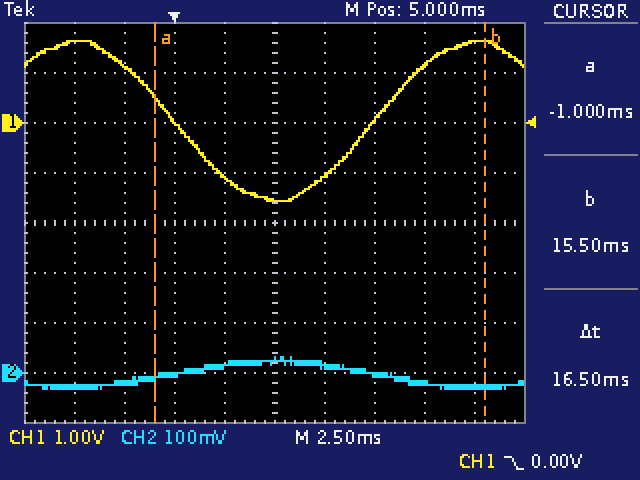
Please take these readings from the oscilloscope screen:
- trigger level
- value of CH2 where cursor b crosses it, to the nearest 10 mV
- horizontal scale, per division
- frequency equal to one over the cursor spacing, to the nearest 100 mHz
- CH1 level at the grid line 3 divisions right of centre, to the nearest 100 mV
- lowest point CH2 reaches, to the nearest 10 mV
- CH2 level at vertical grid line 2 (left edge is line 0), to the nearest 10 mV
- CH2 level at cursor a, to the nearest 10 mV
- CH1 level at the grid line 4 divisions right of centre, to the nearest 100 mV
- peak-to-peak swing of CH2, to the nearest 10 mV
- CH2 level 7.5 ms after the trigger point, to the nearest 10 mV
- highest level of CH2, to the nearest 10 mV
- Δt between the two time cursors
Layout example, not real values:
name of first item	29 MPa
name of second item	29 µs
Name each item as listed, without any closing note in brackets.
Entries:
trigger level	0.00 V
value of CH2 where cursor b crosses it, to the nearest 10 mV	-30 mV
horizontal scale, per division	2.5 ms
frequency equal to one over the cursor spacing, to the nearest 100 mHz	60.6 Hz
CH1 level at the grid line 3 divisions right of centre, to the nearest 100 mV	1.2 V
lowest point CH2 reaches, to the nearest 10 mV	-30 mV
CH2 level at vertical grid line 2 (left edge is line 0), to the nearest 10 mV	-20 mV
CH2 level at cursor a, to the nearest 10 mV	-10 mV
CH1 level at the grid line 4 divisions right of centre, to the nearest 100 mV	1.6 V
peak-to-peak swing of CH2, to the nearest 10 mV	60 mV
CH2 level 7.5 ms after the trigger point, to the nearest 10 mV	20 mV
highest level of CH2, to the nearest 10 mV	30 mV
Δt between the two time cursors	16.5 ms
